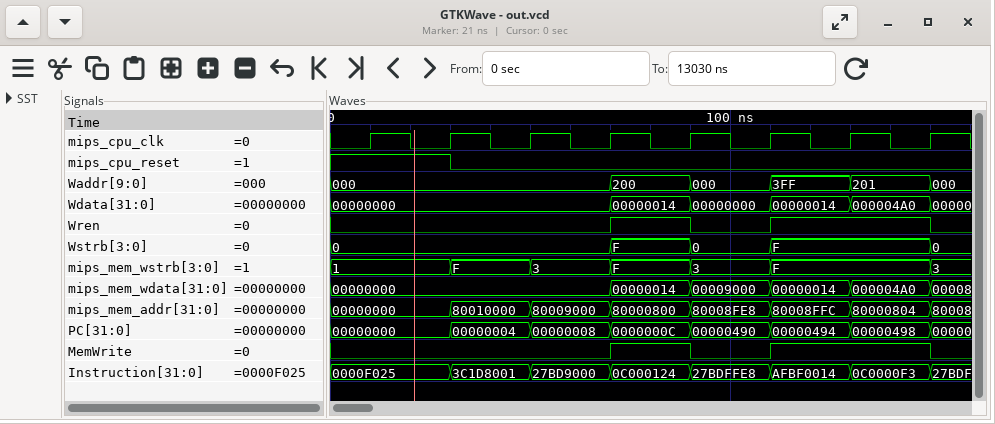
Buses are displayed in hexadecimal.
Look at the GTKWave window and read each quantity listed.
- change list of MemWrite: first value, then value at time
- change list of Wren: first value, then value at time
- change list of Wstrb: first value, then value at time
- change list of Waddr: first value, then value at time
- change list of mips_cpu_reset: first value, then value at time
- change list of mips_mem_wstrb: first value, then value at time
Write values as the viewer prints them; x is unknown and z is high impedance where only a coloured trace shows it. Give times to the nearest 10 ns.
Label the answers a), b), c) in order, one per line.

a) 0, 1 at 70 ns, 0 at 90 ns, 1 at 110 ns, 0 at 150 ns
b) 0, 1 at 70 ns, 0 at 90 ns, 1 at 110 ns, 0 at 150 ns
c) 0, F at 70 ns, 0 at 90 ns, F at 110 ns, 0 at 150 ns
d) 000, 200 at 70 ns, 000 at 90 ns, 3FF at 110 ns, 201 at 130 ns, 000 at 150 ns
e) 1, 0 at 30 ns
f) 1, F at 30 ns, 3 at 50 ns, F at 70 ns, 3 at 90 ns, F at 110 ns, 3 at 150 ns
